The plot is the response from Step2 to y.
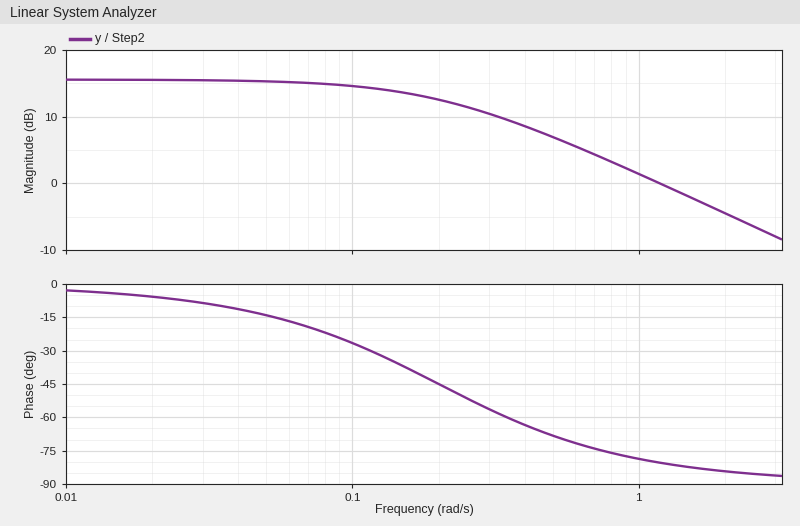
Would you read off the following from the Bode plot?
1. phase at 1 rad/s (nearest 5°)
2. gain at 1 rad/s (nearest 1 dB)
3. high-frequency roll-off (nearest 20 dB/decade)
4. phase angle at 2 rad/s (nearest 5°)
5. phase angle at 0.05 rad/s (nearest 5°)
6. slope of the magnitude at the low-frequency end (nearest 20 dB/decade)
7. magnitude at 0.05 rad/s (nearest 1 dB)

-80°
1 dB
-20 dB/decade
-85°
-15°
0 dB/decade
15 dB
